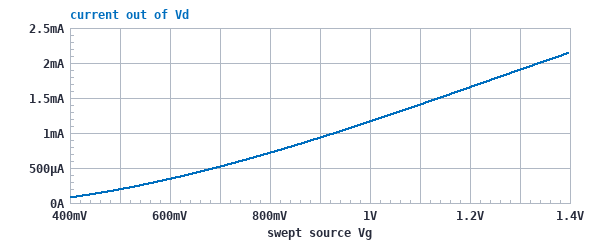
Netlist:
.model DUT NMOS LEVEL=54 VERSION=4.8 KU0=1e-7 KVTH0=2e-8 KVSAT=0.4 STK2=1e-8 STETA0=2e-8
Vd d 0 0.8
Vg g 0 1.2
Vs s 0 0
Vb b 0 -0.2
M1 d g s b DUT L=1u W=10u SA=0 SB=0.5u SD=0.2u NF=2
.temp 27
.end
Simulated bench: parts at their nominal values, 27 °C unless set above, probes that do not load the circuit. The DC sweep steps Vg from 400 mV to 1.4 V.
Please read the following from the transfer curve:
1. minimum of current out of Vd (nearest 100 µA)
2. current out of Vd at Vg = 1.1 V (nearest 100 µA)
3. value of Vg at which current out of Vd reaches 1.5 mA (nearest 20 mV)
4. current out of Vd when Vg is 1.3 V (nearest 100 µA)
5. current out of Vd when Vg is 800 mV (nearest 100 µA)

100 µA
1.4 mA
1.14 V
1.9 mA
700 µA
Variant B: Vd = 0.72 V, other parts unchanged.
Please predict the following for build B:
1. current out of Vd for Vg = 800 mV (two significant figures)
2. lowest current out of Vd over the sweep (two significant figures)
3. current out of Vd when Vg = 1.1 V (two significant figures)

710 µA
80 µA
1.4 mA
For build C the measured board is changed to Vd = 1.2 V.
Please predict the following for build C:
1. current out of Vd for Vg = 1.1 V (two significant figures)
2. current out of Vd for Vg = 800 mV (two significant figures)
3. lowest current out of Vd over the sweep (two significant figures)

1.5 mA
740 µA
85 µA
